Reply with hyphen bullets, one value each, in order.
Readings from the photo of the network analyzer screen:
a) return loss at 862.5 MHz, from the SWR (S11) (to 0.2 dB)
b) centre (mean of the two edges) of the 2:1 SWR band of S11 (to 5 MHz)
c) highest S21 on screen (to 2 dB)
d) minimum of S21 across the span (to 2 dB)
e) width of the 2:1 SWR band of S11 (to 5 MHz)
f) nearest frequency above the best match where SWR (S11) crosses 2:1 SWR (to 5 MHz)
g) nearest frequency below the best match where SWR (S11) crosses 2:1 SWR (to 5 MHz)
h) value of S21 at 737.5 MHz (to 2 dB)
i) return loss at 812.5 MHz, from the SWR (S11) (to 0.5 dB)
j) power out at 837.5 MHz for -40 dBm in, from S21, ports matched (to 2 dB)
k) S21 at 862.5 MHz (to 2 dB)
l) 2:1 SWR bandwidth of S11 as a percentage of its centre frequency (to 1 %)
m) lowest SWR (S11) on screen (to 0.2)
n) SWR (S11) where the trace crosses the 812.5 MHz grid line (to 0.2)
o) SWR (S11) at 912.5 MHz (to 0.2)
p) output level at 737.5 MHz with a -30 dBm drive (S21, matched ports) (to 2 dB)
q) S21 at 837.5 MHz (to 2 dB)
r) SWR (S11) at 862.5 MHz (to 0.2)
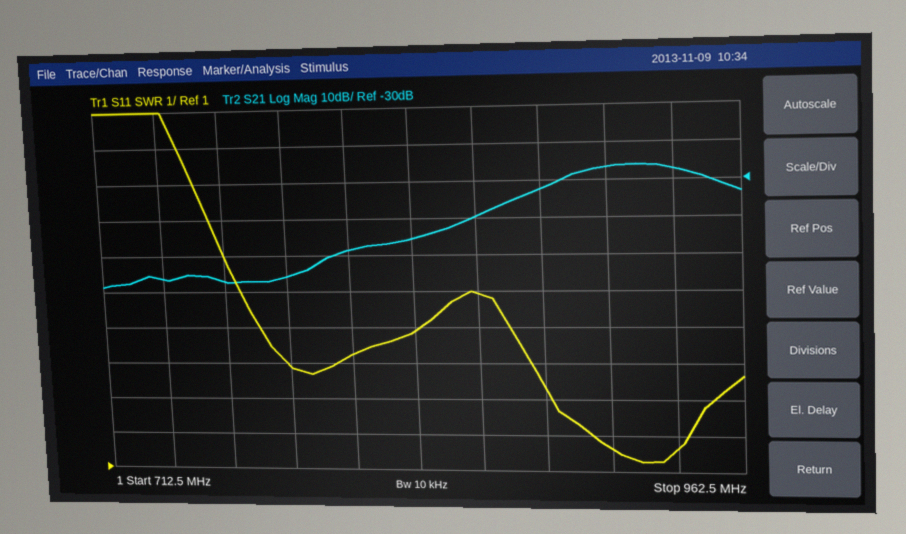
- 3.0 dB
- 925 MHz
- -26 dB
- -58 dB
- 35 MHz
- 940 MHz
- 905 MHz
- -56 dB
- 4.0 dB
- -86 dBm
- -40 dB
- 4 %
- 1.2
- 4.2
- 1.6
- -86 dBm
- -46 dB
- 6.0
